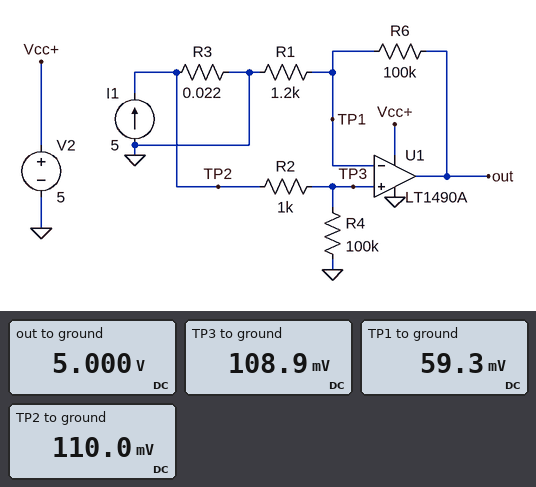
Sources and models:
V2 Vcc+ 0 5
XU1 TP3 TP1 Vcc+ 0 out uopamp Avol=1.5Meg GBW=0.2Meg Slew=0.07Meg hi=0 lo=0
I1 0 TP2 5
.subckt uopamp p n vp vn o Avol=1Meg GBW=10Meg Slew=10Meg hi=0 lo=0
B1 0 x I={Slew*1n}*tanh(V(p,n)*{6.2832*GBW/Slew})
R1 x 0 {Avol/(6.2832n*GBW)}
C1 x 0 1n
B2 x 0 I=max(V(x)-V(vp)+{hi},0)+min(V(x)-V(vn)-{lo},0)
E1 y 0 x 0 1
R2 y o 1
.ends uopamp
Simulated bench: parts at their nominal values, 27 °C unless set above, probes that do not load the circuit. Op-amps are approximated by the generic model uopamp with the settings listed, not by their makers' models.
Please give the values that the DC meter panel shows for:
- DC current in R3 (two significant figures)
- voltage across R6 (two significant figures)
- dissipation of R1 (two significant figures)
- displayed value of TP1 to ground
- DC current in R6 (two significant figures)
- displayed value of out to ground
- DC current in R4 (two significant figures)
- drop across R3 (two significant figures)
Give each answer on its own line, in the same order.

5.0 A
4.9 V
2.9 µW
59.3 mV
49 µA
5.000 V
1.1 µA
110 mV
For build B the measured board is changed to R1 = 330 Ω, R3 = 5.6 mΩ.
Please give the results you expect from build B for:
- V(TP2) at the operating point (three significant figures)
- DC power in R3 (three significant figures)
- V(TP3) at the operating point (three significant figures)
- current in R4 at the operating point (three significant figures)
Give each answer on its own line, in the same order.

28.0 mV
140 mW
27.7 mV
277 nA
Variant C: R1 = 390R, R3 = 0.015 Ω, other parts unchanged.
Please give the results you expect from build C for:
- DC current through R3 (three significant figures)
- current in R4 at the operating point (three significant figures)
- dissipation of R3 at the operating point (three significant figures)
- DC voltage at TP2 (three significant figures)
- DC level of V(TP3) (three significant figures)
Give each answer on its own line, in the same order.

5.00 A
743 nA
375 mW
75.0 mV
74.3 mV
